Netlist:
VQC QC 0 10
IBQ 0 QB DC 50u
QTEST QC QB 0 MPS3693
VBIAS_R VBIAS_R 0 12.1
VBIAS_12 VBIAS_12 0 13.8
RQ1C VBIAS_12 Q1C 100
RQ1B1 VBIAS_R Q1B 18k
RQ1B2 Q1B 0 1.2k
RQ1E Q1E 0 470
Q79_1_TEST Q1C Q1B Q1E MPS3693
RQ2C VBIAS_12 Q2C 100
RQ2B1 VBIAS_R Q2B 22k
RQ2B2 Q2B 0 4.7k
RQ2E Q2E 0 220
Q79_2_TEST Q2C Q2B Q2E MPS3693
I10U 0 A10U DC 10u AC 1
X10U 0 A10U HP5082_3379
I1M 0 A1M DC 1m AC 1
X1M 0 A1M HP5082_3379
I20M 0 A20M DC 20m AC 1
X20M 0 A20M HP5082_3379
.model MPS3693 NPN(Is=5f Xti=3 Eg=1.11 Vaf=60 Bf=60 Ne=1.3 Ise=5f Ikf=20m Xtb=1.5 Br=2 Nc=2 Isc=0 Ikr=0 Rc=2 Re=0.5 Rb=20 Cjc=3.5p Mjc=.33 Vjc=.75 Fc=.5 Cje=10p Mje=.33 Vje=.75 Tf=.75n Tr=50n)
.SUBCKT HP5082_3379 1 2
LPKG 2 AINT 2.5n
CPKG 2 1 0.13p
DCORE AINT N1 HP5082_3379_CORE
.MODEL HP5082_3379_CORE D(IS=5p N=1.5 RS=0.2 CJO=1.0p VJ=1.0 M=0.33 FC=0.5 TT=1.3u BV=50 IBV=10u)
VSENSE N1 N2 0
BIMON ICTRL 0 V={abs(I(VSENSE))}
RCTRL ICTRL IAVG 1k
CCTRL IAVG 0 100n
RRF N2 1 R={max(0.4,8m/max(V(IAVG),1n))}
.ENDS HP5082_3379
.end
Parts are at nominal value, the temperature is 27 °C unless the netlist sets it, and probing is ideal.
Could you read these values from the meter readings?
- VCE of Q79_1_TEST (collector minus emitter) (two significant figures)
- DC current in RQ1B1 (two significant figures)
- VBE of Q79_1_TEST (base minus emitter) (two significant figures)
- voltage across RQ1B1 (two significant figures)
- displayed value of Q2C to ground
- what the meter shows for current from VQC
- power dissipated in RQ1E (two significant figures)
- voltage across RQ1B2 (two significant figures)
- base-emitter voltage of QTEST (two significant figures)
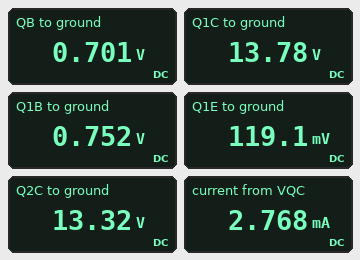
14 V
630 µA
630 mV
11 V
13.32 V
2.768 mA
30 µW
750 mV
700 mV
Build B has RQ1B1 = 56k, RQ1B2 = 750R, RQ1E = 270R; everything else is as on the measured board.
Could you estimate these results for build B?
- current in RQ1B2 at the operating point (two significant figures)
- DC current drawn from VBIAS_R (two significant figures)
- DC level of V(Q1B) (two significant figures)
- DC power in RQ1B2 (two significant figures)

210 µA
680 µA
160 mV
34 µW
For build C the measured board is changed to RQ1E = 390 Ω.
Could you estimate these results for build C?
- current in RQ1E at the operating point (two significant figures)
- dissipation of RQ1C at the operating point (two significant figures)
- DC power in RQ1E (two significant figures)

290 µA
8.3 µW
34 µW
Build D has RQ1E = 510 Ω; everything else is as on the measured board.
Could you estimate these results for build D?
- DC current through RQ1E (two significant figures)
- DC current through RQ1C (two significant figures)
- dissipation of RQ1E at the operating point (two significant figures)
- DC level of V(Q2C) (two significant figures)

240 µA
230 µA
29 µW
13 V
